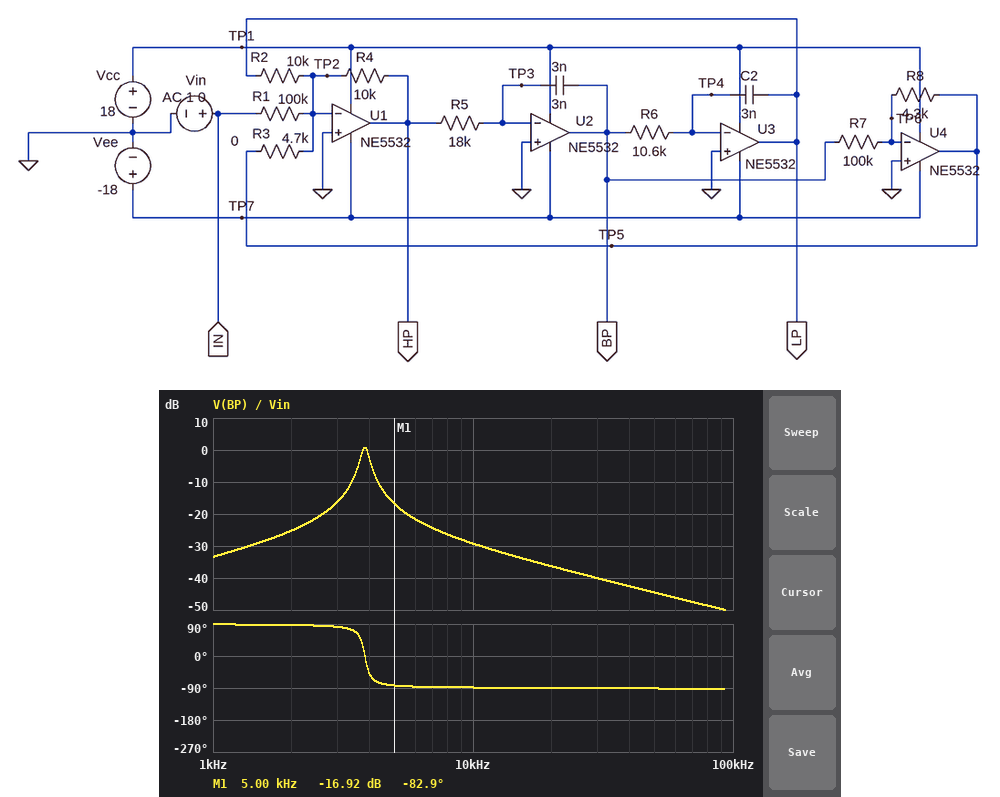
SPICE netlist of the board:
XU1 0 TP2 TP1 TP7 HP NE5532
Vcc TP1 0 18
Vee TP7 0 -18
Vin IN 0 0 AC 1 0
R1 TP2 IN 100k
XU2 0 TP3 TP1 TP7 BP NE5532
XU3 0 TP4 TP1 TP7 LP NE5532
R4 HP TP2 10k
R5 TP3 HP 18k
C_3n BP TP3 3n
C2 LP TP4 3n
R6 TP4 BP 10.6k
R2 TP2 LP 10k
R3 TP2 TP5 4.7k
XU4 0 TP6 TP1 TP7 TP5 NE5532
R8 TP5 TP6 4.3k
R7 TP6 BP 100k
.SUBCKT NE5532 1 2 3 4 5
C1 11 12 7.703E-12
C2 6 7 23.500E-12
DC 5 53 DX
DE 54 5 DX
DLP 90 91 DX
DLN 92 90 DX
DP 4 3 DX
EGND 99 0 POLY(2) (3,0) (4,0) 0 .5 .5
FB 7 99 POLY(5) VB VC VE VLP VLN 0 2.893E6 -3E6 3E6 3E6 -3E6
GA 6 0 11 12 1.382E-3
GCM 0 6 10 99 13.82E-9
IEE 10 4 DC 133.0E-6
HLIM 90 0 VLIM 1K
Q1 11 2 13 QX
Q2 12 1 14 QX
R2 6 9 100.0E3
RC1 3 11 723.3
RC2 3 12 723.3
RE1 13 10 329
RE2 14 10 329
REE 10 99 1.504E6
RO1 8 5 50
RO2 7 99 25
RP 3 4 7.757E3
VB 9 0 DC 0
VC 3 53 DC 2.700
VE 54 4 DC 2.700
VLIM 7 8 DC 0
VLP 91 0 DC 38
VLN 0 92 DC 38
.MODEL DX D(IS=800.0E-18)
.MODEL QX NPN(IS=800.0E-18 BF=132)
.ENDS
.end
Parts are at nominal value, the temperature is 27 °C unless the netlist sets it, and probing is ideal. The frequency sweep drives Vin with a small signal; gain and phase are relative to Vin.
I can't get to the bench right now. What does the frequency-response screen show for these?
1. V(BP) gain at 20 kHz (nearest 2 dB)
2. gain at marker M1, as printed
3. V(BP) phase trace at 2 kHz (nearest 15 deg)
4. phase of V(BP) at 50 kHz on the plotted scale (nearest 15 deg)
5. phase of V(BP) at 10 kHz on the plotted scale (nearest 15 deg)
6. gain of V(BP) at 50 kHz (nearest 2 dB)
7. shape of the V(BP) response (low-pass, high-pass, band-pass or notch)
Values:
-36 dB
-16.92 dB
90 deg
-90 deg
-90 deg
-44 dB
band-pass
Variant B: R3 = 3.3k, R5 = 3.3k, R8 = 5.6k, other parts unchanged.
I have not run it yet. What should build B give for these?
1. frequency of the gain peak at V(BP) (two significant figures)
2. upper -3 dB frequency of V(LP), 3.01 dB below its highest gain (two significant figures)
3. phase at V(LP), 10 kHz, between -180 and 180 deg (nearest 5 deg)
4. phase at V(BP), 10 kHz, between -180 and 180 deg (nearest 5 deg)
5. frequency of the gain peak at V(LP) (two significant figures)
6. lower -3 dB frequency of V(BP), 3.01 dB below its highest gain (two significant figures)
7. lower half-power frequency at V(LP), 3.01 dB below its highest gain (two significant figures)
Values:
9.0 kHz
10 kHz
55 deg
-35 deg
8.8 kHz
7.7 kHz
7.3 kHz
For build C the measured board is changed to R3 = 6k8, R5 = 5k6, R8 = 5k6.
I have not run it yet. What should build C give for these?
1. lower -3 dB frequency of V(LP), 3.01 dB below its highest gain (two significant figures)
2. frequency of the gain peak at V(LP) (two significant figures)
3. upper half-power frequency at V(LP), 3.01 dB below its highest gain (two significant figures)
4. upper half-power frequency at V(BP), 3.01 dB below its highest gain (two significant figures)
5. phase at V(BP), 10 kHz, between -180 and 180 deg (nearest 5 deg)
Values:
6.5 kHz
6.9 kHz
7.2 kHz
7.3 kHz
-80 deg
